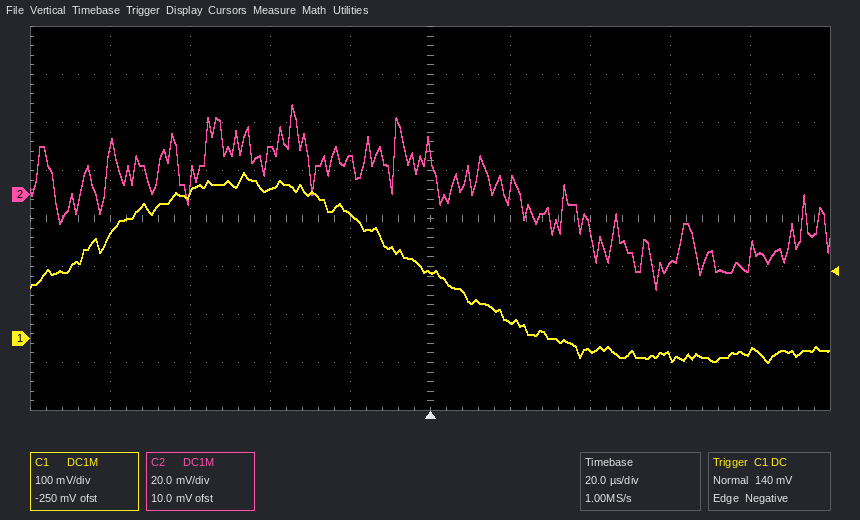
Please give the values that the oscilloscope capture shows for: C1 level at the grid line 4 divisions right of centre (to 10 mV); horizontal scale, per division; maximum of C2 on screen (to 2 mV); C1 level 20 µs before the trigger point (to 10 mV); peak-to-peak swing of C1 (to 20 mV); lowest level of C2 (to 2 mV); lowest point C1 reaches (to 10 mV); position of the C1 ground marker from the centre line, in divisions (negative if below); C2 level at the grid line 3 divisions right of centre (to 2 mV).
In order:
-30 mV
20 µs
38 mV
260 mV
400 mV
-40 mV
-50 mV
-2.5 div
-30 mV
